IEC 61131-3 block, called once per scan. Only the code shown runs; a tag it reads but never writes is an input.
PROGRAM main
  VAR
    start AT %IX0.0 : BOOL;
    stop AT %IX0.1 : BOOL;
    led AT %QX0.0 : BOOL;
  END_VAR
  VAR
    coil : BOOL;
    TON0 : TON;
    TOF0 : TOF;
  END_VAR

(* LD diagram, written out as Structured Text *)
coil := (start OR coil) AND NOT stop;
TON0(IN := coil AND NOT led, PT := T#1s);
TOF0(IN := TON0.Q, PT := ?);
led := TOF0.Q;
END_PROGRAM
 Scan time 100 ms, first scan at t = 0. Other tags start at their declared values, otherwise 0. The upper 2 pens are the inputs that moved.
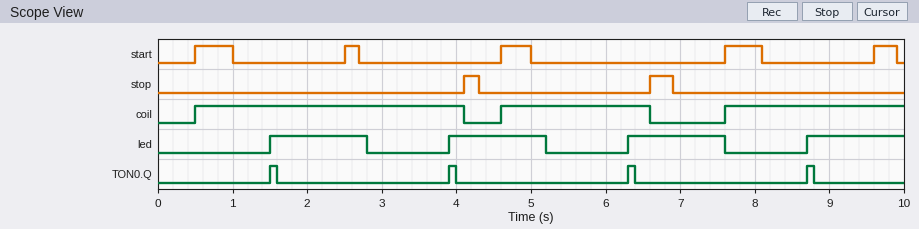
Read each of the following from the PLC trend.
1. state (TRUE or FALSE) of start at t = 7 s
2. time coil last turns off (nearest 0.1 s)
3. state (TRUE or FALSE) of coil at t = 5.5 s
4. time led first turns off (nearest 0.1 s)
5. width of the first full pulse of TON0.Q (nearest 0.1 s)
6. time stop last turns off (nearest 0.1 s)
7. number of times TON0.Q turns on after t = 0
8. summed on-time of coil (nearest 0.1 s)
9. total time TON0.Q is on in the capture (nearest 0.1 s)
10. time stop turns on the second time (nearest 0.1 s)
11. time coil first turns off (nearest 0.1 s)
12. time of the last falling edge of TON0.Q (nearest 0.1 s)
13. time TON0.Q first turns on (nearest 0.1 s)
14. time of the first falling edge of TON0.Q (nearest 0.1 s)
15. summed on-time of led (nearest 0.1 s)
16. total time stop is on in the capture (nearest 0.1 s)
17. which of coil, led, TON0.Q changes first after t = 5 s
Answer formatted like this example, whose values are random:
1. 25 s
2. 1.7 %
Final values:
1. FALSE
2. 6.6 s
3. TRUE
4. 2.8 s
5. 0.1 s
6. 6.9 s
7. 4
8. 8.0 s
9. 0.4 s
10. 6.6 s
11. 4.1 s
12. 8.8 s
13. 1.5 s
14. 1.6 s
15. 5.2 s
16. 0.5 s
17. led
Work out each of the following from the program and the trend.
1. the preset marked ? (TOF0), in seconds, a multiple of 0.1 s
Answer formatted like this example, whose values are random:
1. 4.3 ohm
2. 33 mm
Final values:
1. 1.2 s
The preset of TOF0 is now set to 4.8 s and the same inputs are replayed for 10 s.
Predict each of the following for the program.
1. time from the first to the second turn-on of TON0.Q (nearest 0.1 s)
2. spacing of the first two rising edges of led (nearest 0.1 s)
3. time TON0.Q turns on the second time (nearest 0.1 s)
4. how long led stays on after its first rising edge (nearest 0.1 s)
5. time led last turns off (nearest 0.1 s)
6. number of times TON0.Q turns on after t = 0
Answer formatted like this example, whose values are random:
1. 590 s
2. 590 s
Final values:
1. 7.1 s
2. 7.1 s
3. 8.6 s
4. 4.9 s
5. 6.4 s
6. 2
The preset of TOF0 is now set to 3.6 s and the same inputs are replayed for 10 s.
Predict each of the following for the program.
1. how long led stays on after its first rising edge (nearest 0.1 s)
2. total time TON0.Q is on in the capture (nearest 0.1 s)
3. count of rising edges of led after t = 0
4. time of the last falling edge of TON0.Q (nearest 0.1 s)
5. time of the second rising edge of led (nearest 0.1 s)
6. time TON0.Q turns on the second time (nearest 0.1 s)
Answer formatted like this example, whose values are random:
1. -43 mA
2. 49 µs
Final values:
1. 3.7 s
2. 0.2 s
3. 2
4. 6.4 s
5. 6.3 s
6. 6.3 s
